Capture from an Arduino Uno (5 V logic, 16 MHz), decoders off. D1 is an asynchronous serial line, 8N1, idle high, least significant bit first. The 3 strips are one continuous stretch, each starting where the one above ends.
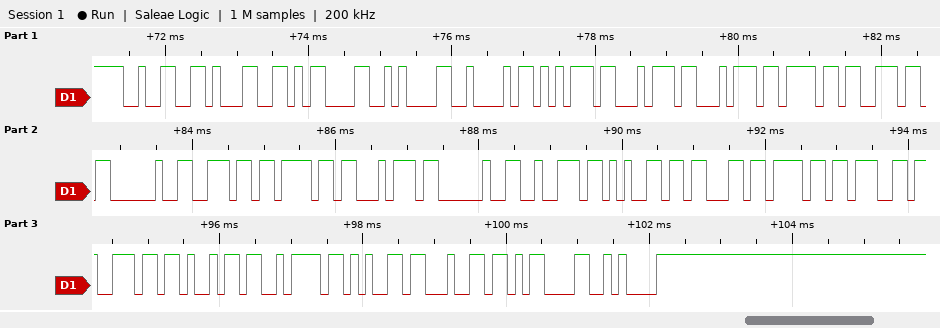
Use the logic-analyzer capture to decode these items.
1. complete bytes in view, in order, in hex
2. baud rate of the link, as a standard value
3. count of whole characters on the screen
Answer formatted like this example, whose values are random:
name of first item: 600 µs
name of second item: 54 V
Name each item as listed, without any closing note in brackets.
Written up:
complete bytes in view, in order, in hex: 32 31 0D 0A 42 75 74 74 6F 6E 20 6E 6F 74 20 72 65 63 6F 67 6E 69 7A 65 64 0D 0A
baud rate of the link, as a standard value: 9600 baud
count of whole characters on the screen: 27
